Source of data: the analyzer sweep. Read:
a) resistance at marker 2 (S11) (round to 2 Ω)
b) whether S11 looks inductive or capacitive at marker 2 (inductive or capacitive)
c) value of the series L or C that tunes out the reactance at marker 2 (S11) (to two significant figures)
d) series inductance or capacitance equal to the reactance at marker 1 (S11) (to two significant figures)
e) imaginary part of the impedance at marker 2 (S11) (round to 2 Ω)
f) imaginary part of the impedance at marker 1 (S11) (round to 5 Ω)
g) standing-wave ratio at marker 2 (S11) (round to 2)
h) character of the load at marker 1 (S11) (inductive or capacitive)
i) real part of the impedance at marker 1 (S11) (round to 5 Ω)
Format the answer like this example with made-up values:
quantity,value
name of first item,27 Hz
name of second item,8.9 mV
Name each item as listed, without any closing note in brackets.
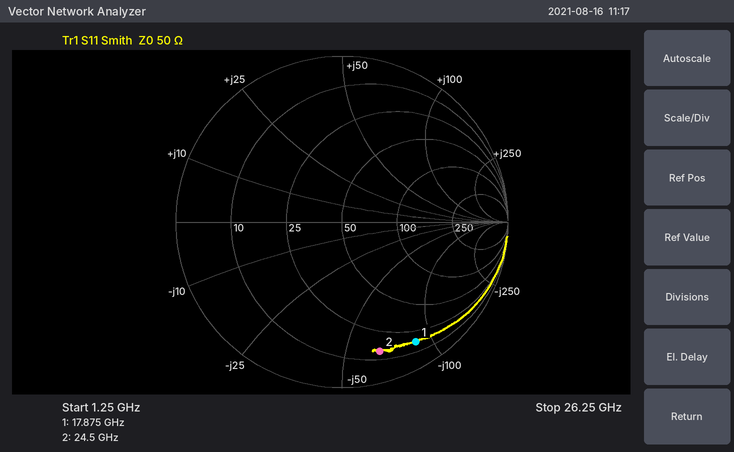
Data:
quantity,value
resistance at marker 2 (S11),14 Ω
whether S11 looks inductive or capacitive at marker 2,capacitive
value of the series L or C that tunes out the reactance at marker 2 (S11),420 pH
series inductance or capacitance equal to the reactance at marker 1 (S11),100 fF
imaginary part of the impedance at marker 2 (S11),-64 Ω
imaginary part of the impedance at marker 1 (S11),-85 Ω
standing-wave ratio at marker 2 (S11),10
character of the load at marker 1 (S11),capacitive
real part of the impedance at marker 1 (S11),15 Ω
